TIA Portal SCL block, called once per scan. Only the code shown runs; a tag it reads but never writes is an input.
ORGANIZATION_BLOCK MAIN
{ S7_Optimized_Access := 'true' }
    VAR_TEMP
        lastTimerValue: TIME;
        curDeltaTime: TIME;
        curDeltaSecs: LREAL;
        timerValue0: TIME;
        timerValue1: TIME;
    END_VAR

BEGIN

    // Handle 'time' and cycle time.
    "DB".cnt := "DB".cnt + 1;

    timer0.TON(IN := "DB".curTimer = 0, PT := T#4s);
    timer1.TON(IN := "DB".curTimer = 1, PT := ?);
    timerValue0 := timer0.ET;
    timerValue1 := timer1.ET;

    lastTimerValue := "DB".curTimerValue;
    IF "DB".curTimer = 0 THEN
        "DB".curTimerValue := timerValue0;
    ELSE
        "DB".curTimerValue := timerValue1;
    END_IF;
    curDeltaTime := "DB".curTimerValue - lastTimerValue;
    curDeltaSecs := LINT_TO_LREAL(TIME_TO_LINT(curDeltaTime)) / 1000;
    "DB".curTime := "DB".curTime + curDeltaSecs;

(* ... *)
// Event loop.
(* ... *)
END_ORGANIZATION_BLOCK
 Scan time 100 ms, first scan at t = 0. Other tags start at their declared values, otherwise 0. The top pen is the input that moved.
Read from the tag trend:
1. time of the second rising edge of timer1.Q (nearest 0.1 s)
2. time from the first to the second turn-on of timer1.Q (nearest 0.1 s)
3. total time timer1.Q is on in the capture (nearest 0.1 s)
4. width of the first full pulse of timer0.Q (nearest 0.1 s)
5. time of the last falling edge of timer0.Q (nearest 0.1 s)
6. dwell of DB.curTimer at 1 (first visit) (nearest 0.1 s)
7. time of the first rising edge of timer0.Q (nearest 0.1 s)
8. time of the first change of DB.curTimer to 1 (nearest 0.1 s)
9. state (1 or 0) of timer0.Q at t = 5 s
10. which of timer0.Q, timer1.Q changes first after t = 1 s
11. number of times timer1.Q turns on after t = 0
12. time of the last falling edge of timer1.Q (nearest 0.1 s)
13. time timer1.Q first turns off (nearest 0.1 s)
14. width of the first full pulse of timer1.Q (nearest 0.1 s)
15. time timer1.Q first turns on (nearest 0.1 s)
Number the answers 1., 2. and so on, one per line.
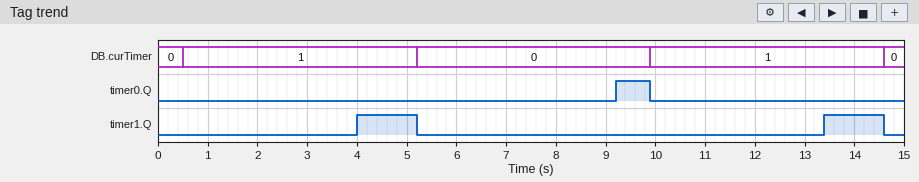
1. 13.4 s
2. 9.4 s
3. 2.4 s
4. 0.7 s
5. 9.9 s
6. 4.7 s
7. 9.2 s
8. 0.5 s
9. 0
10. timer1.Q
11. 2
12. 14.6 s
13. 5.2 s
14. 1.2 s
15. 4.0 s
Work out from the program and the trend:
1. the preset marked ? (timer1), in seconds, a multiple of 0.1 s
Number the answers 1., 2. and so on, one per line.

1. 3.5 s
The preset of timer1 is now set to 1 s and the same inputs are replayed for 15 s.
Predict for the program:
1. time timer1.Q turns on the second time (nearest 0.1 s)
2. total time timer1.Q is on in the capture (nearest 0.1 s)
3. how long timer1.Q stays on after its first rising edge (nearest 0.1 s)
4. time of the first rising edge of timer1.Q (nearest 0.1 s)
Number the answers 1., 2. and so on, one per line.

1. 10.9 s
2. 7.4 s
3. 3.7 s
4. 1.5 s
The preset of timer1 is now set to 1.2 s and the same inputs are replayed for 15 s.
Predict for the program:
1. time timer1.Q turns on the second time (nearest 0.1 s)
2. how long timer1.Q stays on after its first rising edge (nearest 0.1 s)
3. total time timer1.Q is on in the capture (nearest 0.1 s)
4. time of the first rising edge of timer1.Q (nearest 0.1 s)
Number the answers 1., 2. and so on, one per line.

1. 11.1 s
2. 3.5 s
3. 7.0 s
4. 1.7 s
